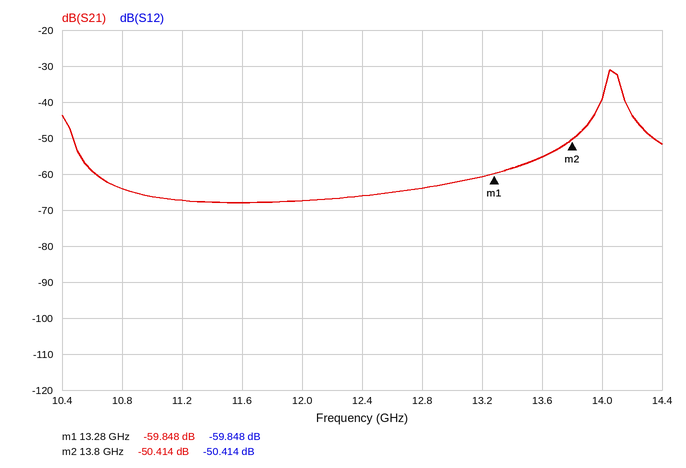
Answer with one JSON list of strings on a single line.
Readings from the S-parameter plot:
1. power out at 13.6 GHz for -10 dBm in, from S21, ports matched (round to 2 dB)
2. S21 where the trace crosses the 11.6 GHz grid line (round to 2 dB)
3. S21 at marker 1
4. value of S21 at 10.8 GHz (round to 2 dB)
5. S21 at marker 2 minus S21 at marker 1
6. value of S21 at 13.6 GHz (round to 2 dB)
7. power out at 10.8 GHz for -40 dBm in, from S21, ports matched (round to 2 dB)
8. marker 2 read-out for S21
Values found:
["-66 dBm", "-68 dB", "-59.848 dB", "-64 dB", "9.434 dB", "-56 dB", "-104 dBm", "-50.414 dB"]
